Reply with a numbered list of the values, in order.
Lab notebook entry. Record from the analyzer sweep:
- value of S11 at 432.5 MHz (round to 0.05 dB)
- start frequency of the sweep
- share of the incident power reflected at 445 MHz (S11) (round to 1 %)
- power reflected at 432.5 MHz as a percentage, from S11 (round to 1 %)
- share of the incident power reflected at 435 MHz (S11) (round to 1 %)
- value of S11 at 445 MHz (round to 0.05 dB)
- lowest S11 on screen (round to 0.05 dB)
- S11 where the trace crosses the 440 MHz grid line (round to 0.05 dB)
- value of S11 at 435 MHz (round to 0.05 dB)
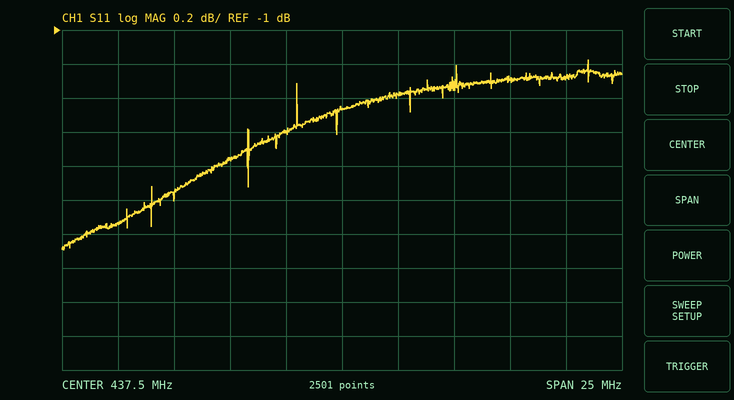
1. -1.75 dB
2. 425 MHz
3. 74 %
4. 67 %
5. 69 %
6. -1.30 dB
7. -2.30 dB
8. -1.40 dB
9. -1.60 dB
